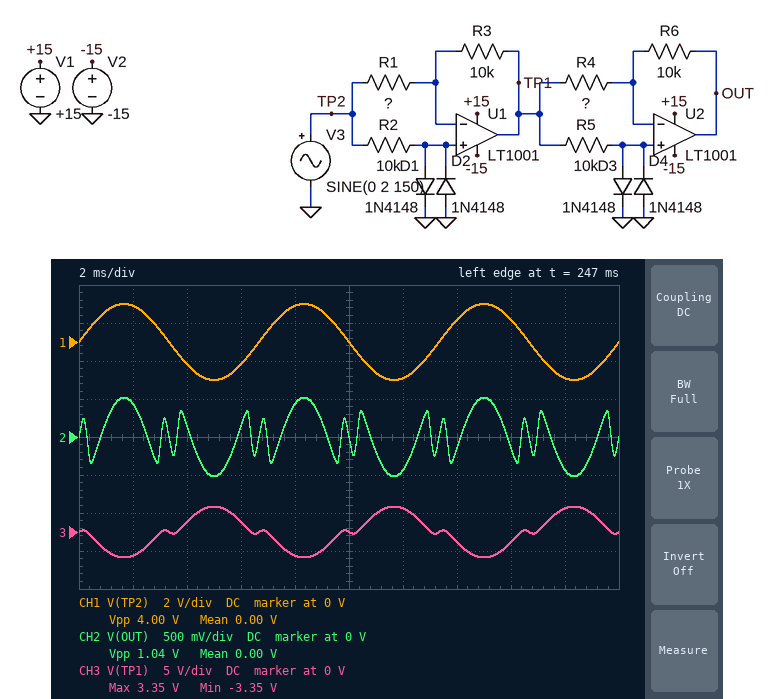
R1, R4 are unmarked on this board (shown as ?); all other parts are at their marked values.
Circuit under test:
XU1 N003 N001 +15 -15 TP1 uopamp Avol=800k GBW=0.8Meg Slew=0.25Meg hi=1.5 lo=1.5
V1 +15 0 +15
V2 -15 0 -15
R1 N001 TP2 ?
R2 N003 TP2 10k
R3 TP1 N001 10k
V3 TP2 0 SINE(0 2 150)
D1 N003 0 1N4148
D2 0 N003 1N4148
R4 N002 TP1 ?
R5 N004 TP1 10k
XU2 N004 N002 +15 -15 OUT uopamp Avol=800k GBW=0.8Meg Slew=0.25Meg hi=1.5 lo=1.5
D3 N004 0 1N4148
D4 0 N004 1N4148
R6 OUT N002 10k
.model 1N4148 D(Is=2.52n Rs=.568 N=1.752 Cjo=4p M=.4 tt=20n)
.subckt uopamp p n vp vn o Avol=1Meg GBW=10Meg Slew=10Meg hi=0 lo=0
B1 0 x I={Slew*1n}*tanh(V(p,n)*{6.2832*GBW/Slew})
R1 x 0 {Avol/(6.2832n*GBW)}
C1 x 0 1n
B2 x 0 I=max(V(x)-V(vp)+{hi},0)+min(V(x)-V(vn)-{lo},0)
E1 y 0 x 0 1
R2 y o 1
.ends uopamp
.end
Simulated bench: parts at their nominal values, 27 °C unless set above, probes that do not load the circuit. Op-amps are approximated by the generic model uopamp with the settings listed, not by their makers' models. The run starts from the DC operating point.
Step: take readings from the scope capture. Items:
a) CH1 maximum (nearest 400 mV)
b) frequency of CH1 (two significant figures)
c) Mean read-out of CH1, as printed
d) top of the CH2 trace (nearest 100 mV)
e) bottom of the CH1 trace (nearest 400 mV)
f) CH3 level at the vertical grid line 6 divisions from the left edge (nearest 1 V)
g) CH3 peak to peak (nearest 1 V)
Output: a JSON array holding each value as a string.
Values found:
["2.0 V", "150 Hz", "0.00 V", "500 mV", "-2.0 V", "3 V", "7 V"]
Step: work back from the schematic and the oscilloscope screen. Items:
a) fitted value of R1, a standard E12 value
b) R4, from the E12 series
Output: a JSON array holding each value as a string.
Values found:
["3.9 kΩ", "27 kΩ"]
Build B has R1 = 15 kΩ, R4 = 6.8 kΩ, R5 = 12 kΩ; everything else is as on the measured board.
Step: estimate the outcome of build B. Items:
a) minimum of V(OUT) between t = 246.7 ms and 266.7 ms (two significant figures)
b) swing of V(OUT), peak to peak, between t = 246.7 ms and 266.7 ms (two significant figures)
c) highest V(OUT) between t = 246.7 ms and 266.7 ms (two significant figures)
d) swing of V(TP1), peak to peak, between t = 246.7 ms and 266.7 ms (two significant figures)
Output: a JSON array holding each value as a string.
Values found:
["-270 mV", "540 mV", "270 mV", "1.0 V"]
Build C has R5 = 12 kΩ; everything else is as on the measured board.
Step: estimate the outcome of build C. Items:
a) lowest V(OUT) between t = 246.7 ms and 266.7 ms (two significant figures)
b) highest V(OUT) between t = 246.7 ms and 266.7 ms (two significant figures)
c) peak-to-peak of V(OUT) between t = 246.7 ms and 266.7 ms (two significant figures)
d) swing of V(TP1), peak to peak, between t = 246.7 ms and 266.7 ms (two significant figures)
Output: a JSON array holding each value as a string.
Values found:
["-530 mV", "530 mV", "1.1 V", "6.7 V"]
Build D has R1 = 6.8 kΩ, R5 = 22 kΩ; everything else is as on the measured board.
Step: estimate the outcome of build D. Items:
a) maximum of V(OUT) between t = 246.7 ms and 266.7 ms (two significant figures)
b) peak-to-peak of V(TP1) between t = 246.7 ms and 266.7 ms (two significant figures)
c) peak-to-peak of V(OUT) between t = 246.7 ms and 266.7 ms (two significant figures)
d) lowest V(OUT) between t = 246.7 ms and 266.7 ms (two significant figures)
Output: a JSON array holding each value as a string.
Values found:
["300 mV", "3.4 V", "610 mV", "-300 mV"]
